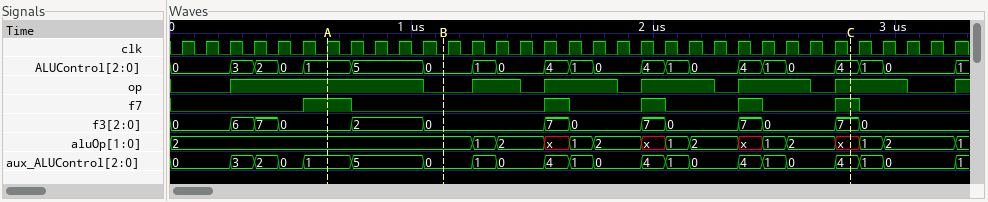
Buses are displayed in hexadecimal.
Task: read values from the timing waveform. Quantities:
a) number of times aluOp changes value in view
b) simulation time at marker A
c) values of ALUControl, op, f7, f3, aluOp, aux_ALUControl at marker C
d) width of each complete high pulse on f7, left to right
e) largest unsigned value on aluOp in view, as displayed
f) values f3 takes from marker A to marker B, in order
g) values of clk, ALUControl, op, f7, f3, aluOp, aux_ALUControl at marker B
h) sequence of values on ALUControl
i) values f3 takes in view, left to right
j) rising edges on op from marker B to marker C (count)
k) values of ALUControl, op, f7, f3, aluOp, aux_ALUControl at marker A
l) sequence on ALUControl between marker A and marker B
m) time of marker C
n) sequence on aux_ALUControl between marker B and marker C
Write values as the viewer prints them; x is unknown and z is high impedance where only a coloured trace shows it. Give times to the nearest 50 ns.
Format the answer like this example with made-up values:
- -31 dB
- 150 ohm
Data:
- 15
- 650 ns
- ALUControl=4, op=1, f7=1, f3=7, aluOp=x, aux_ALUControl=4
- 200 ns, 100 ns, 100 ns, 100 ns, 100 ns
- 2
- 0, 2, 0
- clk=0, ALUControl=0, op=0, f7=0, f3=0, aluOp=2, aux_ALUControl=0
- 0, 3, 2, 0, 1, 5, 0, 1, 0, 4, 1, 0, 4, 1, 0, 4, 1, 0, 4, 1, 0, 1
- 0, 6, 7, 0, 2, 0, 7, 0, 7, 0, 7, 0, 7, 0
- 5
- ALUControl=1, op=1, f7=1, f3=0, aluOp=2, aux_ALUControl=1
- 1, 5, 0
- 2800 ns
- 0, 1, 0, 4, 1, 0, 4, 1, 0, 4, 1, 0, 4
